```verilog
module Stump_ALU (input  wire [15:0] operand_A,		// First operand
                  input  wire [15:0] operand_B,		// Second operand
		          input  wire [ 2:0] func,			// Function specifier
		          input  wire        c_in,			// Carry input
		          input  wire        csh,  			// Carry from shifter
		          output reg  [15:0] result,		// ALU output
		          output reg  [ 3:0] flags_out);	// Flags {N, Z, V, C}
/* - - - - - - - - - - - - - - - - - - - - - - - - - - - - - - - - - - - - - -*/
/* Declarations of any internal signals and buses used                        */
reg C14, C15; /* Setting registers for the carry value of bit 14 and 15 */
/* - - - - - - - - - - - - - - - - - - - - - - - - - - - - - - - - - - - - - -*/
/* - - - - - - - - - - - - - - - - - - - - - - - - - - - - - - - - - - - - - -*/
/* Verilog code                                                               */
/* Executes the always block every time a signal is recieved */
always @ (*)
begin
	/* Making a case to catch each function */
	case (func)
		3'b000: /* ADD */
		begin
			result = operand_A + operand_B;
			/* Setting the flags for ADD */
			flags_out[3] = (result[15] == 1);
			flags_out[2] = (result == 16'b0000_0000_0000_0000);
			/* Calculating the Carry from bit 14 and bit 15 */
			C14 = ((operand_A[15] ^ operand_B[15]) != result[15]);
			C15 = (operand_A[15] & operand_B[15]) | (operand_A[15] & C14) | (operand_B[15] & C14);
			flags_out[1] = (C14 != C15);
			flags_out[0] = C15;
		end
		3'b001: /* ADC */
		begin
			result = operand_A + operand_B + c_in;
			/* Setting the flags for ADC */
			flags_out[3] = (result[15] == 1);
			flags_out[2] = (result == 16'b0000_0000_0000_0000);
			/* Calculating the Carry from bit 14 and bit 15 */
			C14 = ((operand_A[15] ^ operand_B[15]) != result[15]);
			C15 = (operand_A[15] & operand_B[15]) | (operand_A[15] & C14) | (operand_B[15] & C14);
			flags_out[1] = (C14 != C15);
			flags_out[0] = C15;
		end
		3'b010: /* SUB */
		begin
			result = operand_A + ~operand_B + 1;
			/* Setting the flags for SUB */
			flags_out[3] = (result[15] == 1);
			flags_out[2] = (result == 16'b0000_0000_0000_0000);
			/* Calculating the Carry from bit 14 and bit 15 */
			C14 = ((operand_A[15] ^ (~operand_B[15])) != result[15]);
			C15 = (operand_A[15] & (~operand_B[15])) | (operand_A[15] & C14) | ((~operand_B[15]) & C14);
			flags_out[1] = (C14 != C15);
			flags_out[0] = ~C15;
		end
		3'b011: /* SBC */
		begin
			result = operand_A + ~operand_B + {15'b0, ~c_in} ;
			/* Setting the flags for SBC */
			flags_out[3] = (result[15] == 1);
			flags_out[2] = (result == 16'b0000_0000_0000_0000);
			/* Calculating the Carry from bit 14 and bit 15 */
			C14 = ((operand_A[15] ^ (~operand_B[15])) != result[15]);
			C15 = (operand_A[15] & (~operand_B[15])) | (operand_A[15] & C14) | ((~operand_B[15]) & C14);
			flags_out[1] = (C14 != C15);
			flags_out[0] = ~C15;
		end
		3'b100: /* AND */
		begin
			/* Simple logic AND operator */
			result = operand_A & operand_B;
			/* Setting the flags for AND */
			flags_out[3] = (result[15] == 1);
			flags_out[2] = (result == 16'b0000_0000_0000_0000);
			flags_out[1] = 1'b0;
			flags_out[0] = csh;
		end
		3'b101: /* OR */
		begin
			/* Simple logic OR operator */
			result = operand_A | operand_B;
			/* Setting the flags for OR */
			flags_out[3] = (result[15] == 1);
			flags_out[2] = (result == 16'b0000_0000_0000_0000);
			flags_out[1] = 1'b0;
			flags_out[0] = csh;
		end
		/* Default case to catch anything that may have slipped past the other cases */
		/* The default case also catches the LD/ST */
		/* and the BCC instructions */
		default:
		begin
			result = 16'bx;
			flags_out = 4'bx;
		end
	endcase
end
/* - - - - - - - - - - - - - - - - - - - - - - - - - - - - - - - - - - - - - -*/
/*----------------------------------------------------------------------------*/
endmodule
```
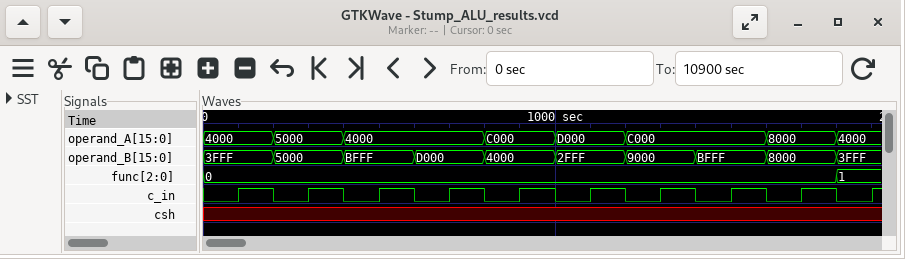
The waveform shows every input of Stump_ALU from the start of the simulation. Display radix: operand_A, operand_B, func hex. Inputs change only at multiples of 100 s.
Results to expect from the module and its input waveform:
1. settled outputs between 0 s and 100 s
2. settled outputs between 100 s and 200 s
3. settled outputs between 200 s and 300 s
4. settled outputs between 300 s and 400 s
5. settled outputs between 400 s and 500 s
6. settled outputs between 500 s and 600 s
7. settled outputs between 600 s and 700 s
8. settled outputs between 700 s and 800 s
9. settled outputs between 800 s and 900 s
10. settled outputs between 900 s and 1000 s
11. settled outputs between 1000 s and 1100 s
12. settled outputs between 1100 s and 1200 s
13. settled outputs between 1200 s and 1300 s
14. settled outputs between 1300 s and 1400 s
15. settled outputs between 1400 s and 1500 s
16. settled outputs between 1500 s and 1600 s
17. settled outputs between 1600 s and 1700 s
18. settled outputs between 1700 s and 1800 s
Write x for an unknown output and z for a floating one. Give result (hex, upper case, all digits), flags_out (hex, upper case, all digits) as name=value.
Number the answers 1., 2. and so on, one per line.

1. result=7FFF, flags_out=0
2. result=7FFF, flags_out=0
3. result=A000, flags_out=A
4. result=A000, flags_out=A
5. result=FFFF, flags_out=8
6. result=FFFF, flags_out=8
7. result=1000, flags_out=1
8. result=1000, flags_out=1
9. result=0000, flags_out=5
10. result=0000, flags_out=5
11. result=FFFF, flags_out=8
12. result=FFFF, flags_out=8
13. result=5000, flags_out=3
14. result=5000, flags_out=3
15. result=7FFF, flags_out=3
16. result=7FFF, flags_out=3
17. result=0000, flags_out=7
18. result=0000, flags_out=7
